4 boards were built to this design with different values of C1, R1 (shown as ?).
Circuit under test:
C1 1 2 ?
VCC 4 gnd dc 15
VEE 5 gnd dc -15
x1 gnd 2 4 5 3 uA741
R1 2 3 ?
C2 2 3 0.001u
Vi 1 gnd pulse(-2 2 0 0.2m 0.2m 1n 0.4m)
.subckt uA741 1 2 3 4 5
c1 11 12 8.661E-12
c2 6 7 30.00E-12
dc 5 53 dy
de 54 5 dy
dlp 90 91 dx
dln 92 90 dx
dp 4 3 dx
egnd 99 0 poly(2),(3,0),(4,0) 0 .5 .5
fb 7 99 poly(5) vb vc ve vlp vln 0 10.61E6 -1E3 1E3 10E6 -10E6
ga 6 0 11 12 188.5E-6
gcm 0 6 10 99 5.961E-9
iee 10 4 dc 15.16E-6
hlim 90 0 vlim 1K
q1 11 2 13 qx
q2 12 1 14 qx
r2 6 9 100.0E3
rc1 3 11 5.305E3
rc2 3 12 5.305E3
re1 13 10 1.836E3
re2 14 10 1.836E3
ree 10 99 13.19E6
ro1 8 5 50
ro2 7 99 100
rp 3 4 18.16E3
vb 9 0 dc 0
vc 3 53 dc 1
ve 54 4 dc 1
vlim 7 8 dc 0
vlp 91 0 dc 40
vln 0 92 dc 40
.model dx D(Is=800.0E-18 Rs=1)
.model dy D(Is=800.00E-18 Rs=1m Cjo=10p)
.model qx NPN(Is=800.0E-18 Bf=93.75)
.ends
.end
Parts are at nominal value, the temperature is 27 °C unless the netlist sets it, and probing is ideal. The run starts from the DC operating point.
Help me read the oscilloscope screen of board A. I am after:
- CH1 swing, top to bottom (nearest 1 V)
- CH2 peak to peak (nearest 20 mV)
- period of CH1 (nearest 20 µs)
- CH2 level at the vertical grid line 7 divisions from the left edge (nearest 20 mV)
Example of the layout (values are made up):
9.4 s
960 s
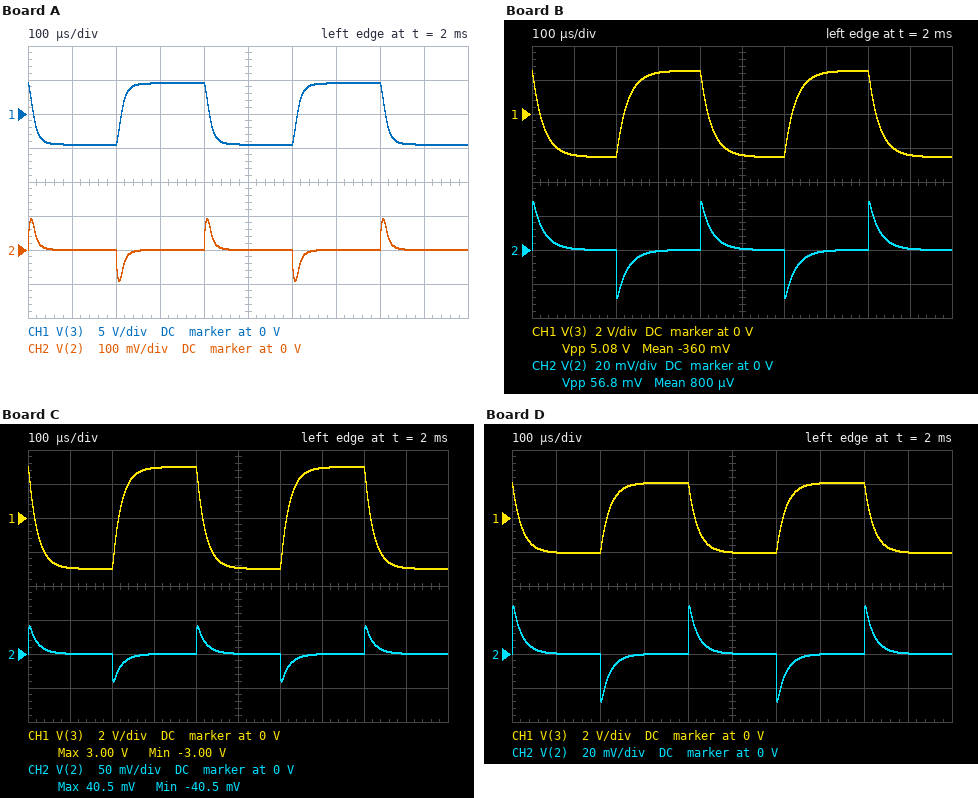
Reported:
9 V
180 mV
400 µs
0 V
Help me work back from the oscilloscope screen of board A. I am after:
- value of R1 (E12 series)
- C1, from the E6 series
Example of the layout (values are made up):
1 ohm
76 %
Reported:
15 kΩ
15 nF
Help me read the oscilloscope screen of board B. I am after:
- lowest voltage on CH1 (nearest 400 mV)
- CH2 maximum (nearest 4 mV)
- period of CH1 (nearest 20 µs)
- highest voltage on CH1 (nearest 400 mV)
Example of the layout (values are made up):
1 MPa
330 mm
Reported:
-2.4 V
28 mV
400 µs
2.4 V
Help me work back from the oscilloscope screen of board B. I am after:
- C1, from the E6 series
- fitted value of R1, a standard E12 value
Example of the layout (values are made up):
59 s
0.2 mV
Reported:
4.7 nF
27 kΩ
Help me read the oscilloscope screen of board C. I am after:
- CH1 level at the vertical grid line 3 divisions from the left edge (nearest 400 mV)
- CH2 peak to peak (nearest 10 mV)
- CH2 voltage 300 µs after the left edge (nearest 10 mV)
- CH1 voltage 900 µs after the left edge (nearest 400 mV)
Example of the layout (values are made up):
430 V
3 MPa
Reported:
2.8 V
80 mV
0 V
-2.8 V
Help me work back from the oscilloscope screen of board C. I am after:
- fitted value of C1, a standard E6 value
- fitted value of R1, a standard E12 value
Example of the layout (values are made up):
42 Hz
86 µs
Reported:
6.8 nF
22 kΩ
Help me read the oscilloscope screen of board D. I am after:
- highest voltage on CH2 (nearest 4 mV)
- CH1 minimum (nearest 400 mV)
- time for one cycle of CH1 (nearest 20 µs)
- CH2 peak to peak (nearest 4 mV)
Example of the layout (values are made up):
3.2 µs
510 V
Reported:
28 mV
-2.0 V
400 µs
56 mV
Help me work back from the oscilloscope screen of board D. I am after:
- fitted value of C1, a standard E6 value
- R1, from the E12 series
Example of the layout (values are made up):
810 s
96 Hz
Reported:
4.7 nF
22 kΩ
